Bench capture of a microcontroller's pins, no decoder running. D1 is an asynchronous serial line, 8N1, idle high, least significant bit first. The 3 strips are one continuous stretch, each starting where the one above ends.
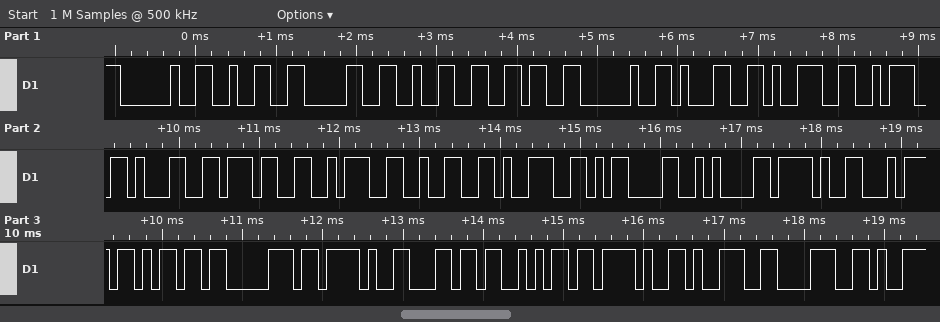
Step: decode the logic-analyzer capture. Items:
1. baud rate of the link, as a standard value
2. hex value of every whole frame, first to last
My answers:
9600 baud
0x20 0x32 0x30 0x32 0x36 0x20 0x31 0x39 0x3A 0x31 0x37 0x3A 0x32 0x39 0x0D 0x0A 0x2F 0x74 0x6D 0x70 0x2F 0x6C 0x6A 0x2F 0x39 0x38
